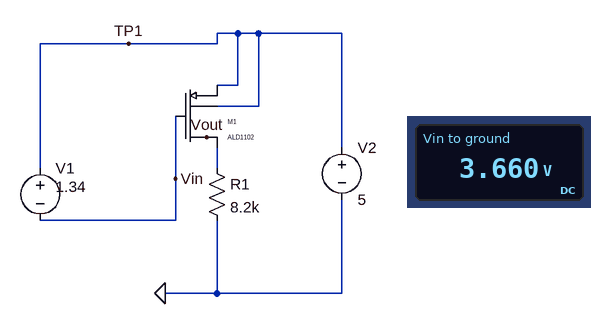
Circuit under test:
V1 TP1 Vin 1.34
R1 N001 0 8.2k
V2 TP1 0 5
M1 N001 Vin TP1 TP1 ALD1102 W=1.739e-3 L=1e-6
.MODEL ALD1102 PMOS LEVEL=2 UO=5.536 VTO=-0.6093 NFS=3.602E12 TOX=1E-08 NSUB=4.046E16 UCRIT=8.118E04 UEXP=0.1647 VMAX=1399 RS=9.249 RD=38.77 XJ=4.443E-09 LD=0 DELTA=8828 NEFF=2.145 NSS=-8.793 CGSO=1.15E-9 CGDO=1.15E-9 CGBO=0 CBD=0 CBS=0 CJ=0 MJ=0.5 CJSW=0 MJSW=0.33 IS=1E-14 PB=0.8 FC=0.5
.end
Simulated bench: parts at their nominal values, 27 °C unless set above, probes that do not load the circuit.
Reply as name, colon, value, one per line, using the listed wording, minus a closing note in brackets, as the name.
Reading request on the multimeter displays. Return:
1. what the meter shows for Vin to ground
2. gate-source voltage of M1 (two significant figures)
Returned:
what the meter shows for Vin to ground: 3.660 V
gate-source voltage of M1: -1.3 V
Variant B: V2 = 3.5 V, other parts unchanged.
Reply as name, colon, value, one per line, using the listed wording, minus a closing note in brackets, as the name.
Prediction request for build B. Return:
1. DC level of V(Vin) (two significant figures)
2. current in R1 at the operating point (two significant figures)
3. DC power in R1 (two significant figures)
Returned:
DC level of V(Vin): 2.2 V
current in R1 at the operating point: 390 µA
DC power in R1: 1.2 mW
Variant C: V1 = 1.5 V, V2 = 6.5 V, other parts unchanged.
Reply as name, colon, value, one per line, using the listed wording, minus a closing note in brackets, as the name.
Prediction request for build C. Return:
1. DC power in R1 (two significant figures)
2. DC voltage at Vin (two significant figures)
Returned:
DC power in R1: 4.1 mW
DC voltage at Vin: 5.0 V
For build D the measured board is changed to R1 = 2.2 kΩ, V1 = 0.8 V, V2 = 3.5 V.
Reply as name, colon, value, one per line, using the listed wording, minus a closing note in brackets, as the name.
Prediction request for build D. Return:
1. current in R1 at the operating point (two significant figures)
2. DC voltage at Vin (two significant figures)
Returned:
current in R1 at the operating point: 20 µA
DC voltage at Vin: 2.7 V
